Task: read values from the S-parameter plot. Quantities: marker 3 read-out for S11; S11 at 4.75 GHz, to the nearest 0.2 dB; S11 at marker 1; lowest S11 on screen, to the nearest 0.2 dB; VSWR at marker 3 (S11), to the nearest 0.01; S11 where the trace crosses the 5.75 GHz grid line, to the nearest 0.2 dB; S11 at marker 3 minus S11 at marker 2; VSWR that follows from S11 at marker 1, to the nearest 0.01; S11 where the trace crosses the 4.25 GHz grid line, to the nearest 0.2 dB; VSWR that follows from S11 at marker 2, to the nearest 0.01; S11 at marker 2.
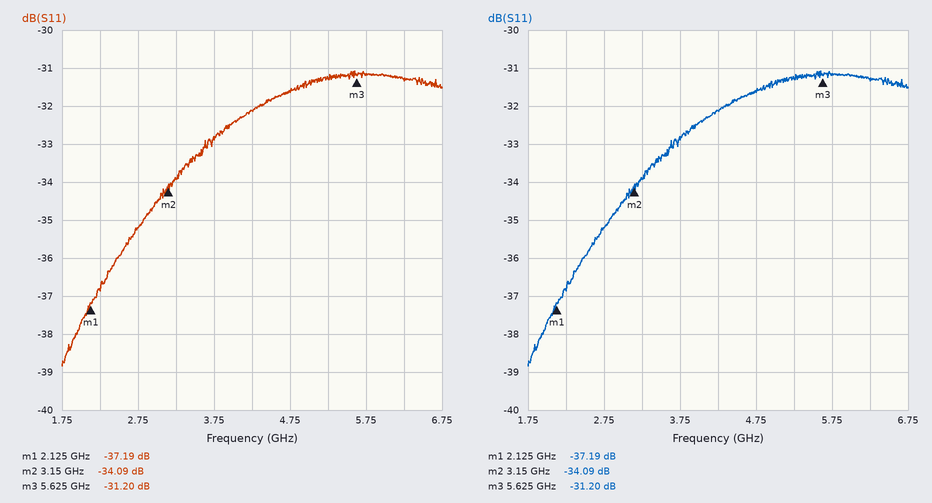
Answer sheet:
-31.20 dB
-31.6 dB
-37.19 dB
-38.8 dB
1.06
-31.2 dB
2.89 dB
1.03
-32.2 dB
1.04
-34.09 dB
